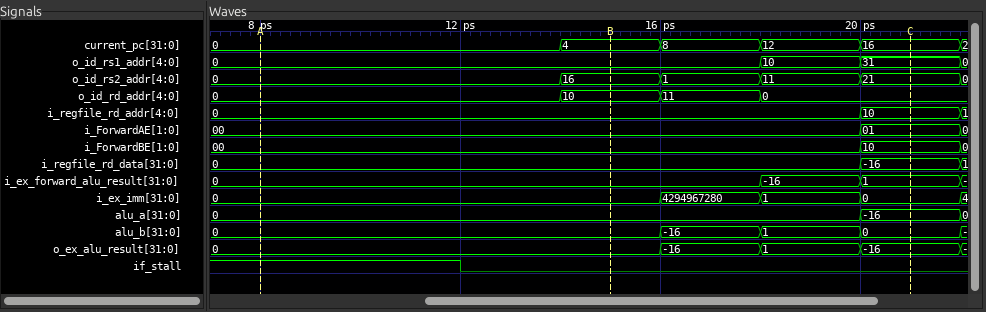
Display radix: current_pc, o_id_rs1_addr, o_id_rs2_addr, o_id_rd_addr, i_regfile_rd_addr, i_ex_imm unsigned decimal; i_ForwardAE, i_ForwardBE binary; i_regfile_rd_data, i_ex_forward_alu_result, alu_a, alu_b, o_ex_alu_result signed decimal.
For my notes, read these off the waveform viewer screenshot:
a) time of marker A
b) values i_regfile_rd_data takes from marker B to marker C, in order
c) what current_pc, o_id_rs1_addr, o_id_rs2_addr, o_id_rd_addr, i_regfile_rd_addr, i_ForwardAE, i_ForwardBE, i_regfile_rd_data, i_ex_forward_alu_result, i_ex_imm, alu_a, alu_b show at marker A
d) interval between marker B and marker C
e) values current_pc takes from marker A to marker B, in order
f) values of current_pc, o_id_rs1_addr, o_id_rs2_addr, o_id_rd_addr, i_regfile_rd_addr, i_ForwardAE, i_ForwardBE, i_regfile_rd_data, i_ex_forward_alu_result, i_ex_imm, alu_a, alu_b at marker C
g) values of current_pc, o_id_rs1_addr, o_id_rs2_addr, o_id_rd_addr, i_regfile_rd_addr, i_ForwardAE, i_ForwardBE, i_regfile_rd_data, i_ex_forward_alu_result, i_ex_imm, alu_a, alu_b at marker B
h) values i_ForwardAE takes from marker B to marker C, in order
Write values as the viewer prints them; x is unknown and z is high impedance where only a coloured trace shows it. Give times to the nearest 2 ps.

8 ps
0, -16
current_pc=0, o_id_rs1_addr=0, o_id_rs2_addr=0, o_id_rd_addr=0, i_regfile_rd_addr=0, i_ForwardAE=00, i_ForwardBE=00, i_regfile_rd_data=0, i_ex_forward_alu_result=0, i_ex_imm=0, alu_a=0, alu_b=0
6 ps
0, 4
current_pc=16, o_id_rs1_addr=31, o_id_rs2_addr=21, o_id_rd_addr=0, i_regfile_rd_addr=10, i_ForwardAE=01, i_ForwardBE=10, i_regfile_rd_data=-16, i_ex_forward_alu_result=1, i_ex_imm=0, alu_a=-16, alu_b=0
current_pc=4, o_id_rs1_addr=0, o_id_rs2_addr=16, o_id_rd_addr=10, i_regfile_rd_addr=0, i_ForwardAE=00, i_ForwardBE=00, i_regfile_rd_data=0, i_ex_forward_alu_result=0, i_ex_imm=0, alu_a=0, alu_b=0
00, 01
